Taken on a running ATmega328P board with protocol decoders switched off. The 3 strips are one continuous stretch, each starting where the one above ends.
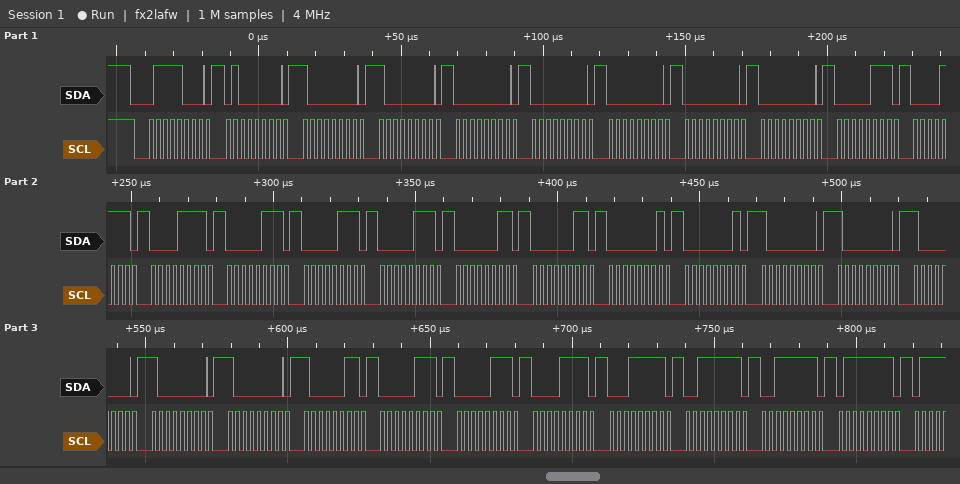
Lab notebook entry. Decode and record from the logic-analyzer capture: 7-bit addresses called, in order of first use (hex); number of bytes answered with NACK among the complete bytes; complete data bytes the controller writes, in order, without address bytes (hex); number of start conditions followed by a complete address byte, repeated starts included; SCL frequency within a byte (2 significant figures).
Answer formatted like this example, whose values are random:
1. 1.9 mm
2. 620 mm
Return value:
1. 0x3C
2. 0
3. 40 80 80 00 00 00 00 00 07 0F 0F 07 07 07 03 03 01 01 80 80 80 80 80 83 07 07 0F 1F 3F 3F 7F
4. 1
5. 400 kHz
